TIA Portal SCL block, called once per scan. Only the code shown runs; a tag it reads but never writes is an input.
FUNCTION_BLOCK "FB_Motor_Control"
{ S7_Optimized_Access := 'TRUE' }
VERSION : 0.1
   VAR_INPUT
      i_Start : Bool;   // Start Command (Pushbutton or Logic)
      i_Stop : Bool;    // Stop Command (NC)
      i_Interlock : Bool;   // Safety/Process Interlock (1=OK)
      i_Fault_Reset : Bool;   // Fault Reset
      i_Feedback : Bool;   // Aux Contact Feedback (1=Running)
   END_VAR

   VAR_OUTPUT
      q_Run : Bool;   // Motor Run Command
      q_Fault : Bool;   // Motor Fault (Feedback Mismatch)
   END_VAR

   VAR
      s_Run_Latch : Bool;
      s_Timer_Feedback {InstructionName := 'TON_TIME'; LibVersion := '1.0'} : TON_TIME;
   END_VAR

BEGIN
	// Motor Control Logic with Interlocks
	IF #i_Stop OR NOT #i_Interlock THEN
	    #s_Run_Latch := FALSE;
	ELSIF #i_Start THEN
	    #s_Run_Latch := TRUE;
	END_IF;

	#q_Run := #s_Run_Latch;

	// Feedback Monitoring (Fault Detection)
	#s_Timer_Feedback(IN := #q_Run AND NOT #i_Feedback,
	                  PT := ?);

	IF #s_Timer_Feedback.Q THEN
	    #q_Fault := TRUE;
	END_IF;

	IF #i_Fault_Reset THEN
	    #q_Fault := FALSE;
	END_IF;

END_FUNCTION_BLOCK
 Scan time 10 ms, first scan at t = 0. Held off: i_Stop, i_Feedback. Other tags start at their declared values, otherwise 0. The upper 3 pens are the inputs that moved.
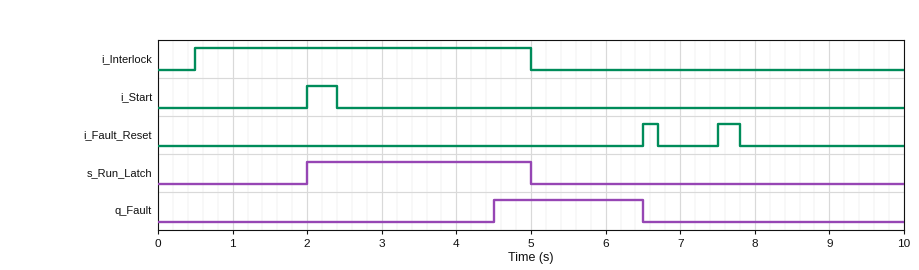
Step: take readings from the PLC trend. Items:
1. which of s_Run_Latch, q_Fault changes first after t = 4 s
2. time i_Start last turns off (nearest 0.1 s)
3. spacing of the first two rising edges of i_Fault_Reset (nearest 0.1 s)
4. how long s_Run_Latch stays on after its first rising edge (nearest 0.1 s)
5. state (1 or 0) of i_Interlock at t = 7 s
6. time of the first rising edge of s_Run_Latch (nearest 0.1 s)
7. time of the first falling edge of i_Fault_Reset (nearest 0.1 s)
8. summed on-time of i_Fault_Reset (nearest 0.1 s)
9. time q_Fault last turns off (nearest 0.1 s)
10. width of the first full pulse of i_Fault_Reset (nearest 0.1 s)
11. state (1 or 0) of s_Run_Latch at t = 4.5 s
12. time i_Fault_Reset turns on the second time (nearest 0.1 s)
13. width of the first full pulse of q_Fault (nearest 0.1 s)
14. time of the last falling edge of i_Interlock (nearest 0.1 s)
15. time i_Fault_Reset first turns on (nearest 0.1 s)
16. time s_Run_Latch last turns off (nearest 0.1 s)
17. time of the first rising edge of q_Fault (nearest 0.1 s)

q_Fault
2.4 s
1.0 s
3.0 s
0
2.0 s
6.7 s
0.5 s
6.5 s
0.2 s
1
7.5 s
2.0 s
5.0 s
6.5 s
5.0 s
4.5 s
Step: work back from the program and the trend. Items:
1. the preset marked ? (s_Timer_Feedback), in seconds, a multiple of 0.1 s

2.5 s
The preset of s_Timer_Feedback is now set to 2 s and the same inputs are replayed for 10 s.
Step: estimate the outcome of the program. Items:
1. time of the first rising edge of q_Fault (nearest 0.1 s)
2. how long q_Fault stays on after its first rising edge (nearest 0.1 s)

4.0 s
2.5 s
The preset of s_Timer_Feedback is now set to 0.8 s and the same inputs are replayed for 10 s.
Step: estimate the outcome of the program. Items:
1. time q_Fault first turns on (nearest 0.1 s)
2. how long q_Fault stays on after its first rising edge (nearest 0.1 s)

2.8 s
3.7 s
